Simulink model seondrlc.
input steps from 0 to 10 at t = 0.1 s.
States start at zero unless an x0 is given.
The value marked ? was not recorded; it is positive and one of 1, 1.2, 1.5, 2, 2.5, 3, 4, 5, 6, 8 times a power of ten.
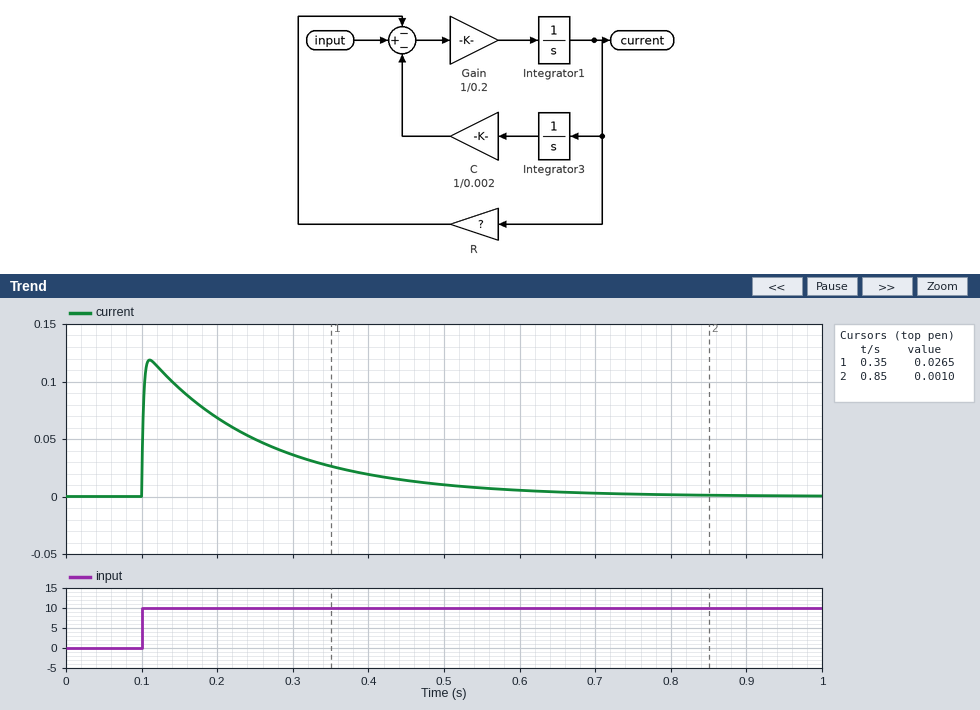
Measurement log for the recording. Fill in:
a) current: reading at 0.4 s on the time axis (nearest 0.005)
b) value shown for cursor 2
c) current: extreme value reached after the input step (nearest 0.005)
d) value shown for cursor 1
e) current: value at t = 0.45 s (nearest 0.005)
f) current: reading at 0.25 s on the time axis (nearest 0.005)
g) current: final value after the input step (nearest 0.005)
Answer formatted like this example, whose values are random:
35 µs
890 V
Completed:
0.020
0.0010
0.120
0.0265
0.015
0.050
0.000
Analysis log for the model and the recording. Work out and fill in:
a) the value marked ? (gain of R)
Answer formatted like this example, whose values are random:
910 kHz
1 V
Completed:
80
